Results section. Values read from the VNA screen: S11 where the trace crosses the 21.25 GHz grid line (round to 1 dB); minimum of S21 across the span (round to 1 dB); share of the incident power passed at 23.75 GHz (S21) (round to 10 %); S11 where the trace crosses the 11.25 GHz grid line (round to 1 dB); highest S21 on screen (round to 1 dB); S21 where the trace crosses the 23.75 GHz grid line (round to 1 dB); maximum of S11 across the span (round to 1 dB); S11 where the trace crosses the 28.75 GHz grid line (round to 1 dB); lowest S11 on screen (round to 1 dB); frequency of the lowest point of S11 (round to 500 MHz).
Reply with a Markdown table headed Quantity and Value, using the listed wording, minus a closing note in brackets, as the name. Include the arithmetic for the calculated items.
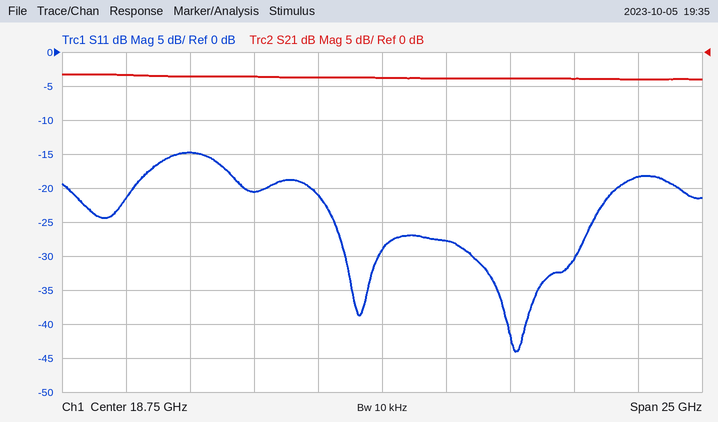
| Quantity | Value |
|---|---|
| S11 where the trace crosses the 21.25 GHz grid line | -28 dB |
| minimum of S21 across the span | -4 dB |
| share of the incident power passed at 23.75 GHz (S21) | 10^(-4/10) ≈ 40 % |
| S11 where the trace crosses the 11.25 GHz grid line | -15 dB |
| highest S21 on screen | -3 dB |
| S21 where the trace crosses the 23.75 GHz grid line | -4 dB |
| maximum of S11 across the span | -15 dB |
| S11 where the trace crosses the 28.75 GHz grid line | -18 dB |
| lowest S11 on screen | -44 dB |
| frequency of the lowest point of S11 | 24.0 GHz |
